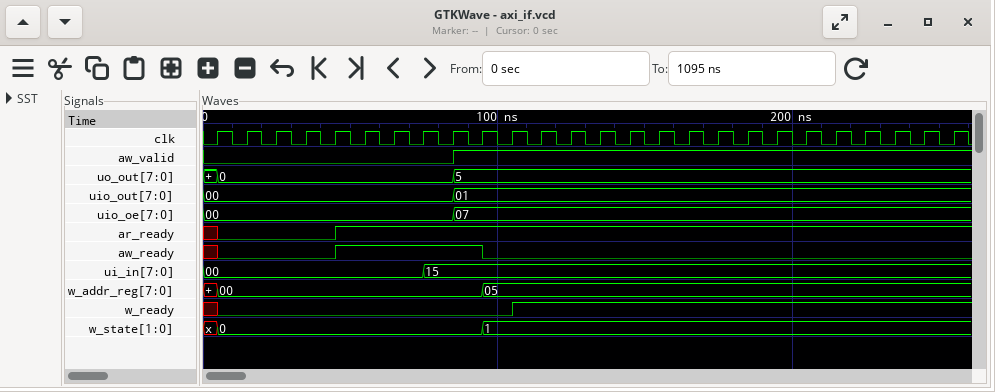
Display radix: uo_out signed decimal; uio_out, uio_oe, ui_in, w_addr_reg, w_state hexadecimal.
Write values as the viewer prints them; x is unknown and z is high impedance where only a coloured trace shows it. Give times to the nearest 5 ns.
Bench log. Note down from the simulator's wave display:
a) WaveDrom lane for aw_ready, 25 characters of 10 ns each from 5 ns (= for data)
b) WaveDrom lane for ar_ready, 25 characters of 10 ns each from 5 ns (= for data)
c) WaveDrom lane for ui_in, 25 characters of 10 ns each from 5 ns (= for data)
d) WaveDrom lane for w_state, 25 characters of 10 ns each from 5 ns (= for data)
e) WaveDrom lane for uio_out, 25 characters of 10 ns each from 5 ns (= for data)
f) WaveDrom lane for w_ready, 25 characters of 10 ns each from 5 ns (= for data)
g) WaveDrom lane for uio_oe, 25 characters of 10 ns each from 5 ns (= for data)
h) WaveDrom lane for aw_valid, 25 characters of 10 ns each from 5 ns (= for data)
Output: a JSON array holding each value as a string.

["{name: 'aw_ready', wave: '0...1....0...............'}", "{name: 'ar_ready', wave: '0...1....................'}", "{name: 'ui_in', wave: '=......=.................', data: '00 15'}", "{name: 'w_state', wave: '=........=...............', data: '0 1'}", "{name: 'uio_out', wave: '=.......=................', data: '00 01'}", "{name: 'w_ready', wave: '0.........1..............'}", "{name: 'uio_oe', wave: '=.......=................', data: '00 07'}", "{name: 'aw_valid', wave: '0.......1................'}"]
